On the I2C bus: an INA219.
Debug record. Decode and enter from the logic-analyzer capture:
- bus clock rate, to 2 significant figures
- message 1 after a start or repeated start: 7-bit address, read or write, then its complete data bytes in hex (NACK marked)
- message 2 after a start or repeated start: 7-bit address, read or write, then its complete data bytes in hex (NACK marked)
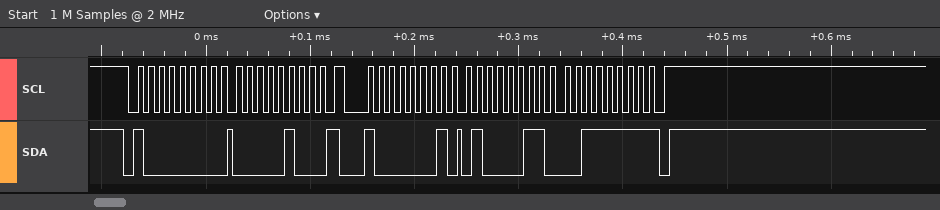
100 kHz
0x40 write: 04
0x40 read: 43 3F NACK
